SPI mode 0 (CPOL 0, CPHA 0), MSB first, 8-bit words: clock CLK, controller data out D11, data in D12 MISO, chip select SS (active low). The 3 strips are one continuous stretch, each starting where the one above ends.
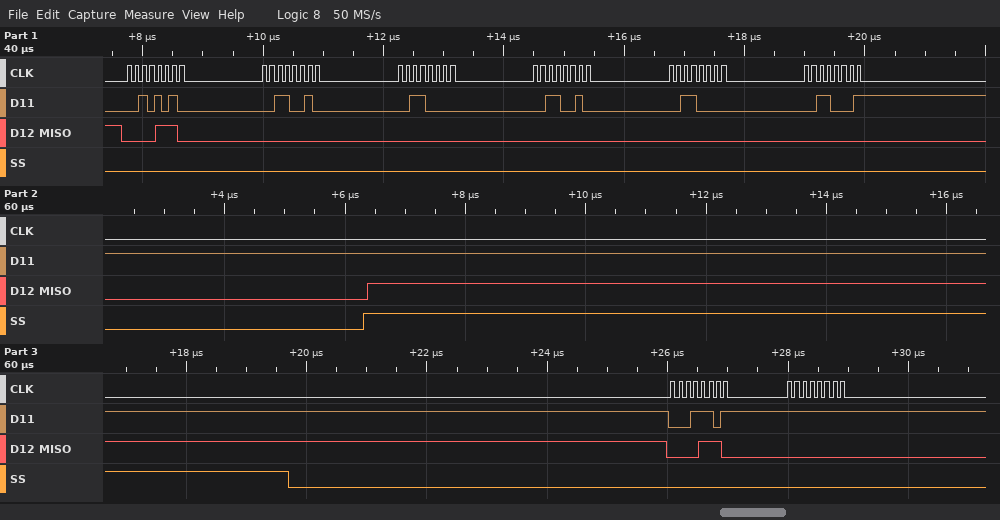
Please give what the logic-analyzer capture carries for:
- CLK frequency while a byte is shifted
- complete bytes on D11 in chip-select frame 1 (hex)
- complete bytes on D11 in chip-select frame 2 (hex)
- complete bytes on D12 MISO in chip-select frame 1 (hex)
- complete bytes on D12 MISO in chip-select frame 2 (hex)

8 MHz
2A 32 30 32 30 31
1D FF
0E 00 00 00 00 00
0E 00
